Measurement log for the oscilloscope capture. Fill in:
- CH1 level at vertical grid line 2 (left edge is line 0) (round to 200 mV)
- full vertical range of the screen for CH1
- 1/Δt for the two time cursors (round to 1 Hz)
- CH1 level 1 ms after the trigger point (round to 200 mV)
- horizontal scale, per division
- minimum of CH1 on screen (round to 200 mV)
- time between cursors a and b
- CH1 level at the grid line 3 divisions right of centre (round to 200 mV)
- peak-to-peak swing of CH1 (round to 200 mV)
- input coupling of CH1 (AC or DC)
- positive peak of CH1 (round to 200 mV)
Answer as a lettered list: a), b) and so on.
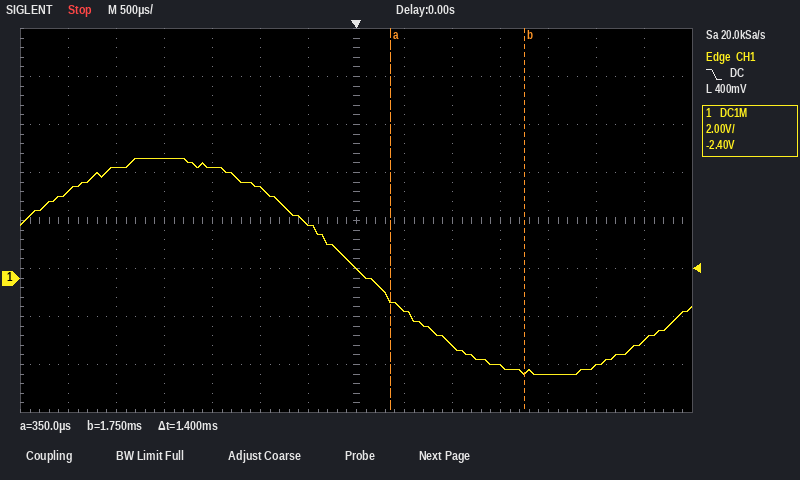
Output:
a) 4.6 V
b) 16 V
c) 714 Hz
d) -2.8 V
e) 500 µs
f) -4.0 V
g) 1.4 ms
h) -3.6 V
i) 9.0 V
j) DC
k) 5.0 V
